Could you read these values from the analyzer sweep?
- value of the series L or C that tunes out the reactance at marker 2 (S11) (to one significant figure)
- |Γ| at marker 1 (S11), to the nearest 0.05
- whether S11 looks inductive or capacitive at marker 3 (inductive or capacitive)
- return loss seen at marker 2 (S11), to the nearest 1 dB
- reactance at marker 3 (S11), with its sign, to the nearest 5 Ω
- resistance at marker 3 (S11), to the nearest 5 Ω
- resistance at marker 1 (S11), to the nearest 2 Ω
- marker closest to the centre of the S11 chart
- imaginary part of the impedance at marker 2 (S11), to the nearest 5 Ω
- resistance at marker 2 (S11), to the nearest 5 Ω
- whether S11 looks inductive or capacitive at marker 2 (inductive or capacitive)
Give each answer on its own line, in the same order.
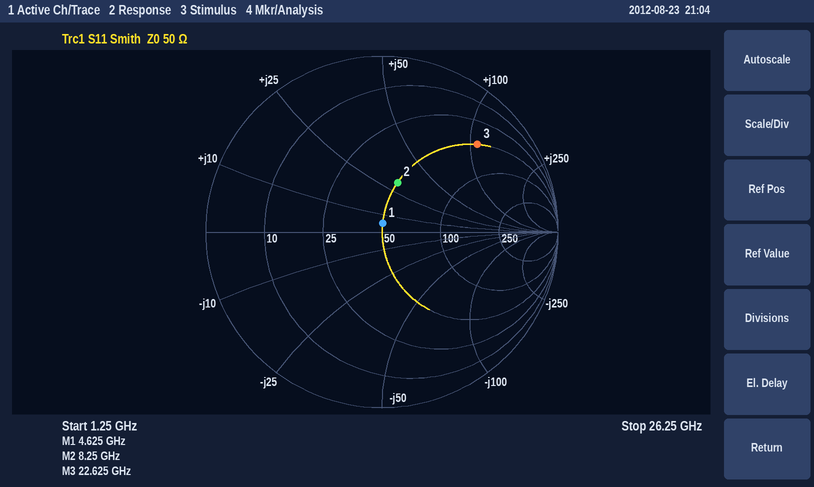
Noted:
600 fF
0.05
inductive
11 dB
+110 Ω
50 Ω
50 Ω
marker 1
+30 Ω
50 Ω
inductive
